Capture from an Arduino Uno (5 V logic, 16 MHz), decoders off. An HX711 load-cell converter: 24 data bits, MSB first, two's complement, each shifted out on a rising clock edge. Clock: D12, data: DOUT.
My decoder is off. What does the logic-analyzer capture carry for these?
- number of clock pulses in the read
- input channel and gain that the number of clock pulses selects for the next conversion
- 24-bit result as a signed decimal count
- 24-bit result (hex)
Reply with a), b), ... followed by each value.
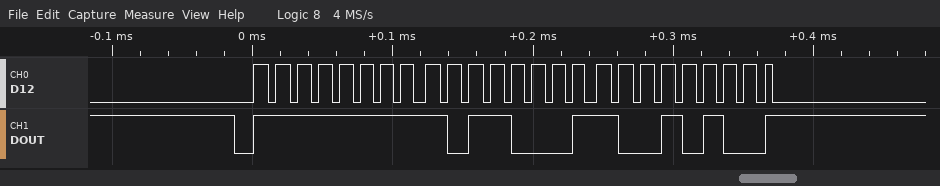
a) 25
b) channel A, gain 128
c) -20076
d) 0xFFB194
